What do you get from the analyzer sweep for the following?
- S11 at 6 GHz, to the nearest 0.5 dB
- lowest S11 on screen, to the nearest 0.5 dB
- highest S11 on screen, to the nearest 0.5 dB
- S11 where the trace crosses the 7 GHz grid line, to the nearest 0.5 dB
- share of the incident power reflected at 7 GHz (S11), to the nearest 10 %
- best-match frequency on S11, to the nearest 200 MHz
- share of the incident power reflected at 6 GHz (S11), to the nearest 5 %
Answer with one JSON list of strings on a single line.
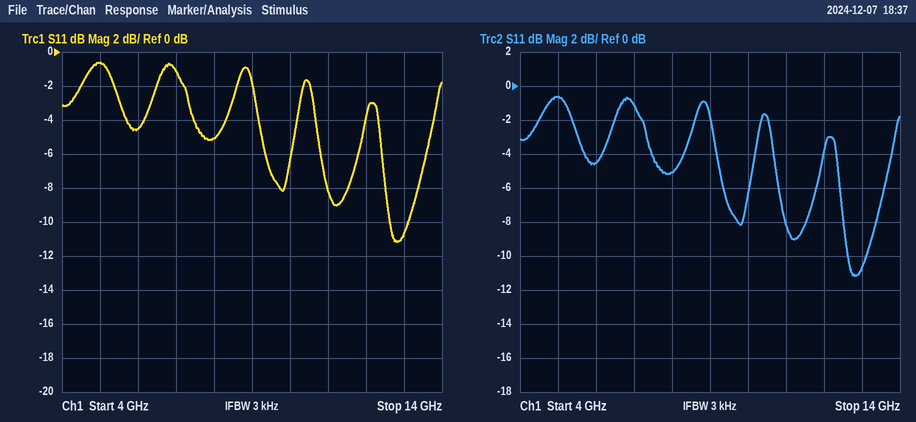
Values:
["-4.5 dB", "-11.0 dB", "-0.5 dB", "-1.0 dB", "80 %", "12.8 GHz", "35 %"]
